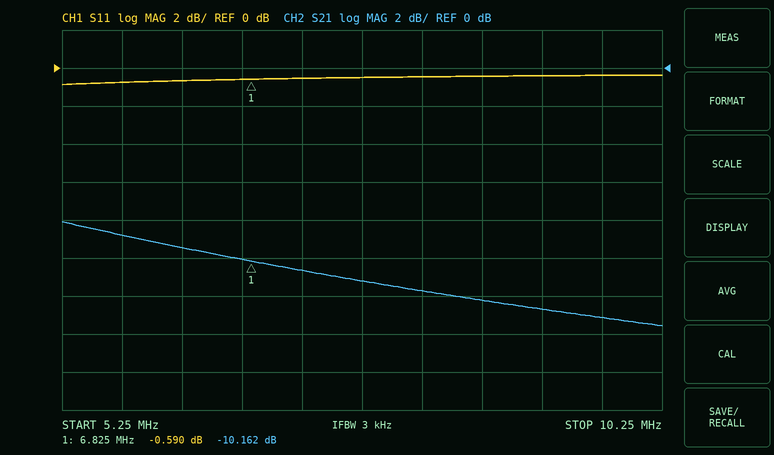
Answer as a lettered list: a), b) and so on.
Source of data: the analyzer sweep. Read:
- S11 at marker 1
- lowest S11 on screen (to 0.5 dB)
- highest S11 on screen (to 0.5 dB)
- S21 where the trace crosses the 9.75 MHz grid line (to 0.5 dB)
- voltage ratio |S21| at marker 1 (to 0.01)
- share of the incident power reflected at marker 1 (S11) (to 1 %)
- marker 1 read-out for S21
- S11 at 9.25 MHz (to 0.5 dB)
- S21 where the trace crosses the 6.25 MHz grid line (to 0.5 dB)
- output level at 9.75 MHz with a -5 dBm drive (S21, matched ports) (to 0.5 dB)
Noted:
a) -0.590 dB
b) -1.0 dB
c) -0.5 dB
d) -13.0 dB
e) 0.31
f) 87 %
g) -10.162 dB
h) -0.5 dB
i) -9.5 dB
j) -18.0 dBm
